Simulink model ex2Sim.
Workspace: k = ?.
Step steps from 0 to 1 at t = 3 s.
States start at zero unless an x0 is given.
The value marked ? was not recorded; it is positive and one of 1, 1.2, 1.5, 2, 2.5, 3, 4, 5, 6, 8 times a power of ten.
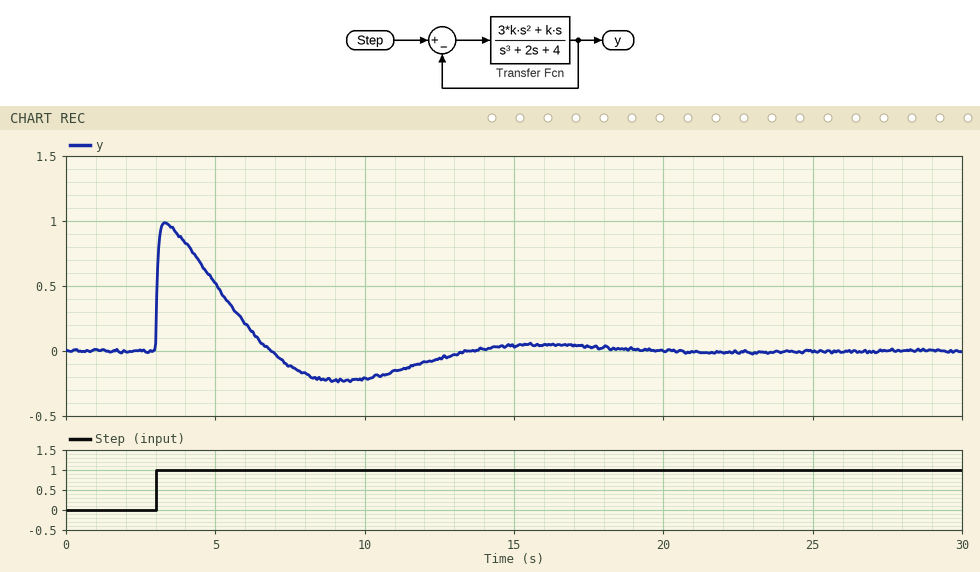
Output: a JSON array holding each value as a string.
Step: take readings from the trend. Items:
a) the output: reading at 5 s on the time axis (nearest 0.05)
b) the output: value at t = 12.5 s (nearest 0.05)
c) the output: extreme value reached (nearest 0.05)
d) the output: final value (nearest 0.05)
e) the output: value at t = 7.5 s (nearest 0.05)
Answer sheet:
["0.50", "-0.05", "1.00", "0.00", "-0.10"]
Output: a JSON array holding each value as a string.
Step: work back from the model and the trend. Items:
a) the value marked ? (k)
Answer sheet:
["5"]
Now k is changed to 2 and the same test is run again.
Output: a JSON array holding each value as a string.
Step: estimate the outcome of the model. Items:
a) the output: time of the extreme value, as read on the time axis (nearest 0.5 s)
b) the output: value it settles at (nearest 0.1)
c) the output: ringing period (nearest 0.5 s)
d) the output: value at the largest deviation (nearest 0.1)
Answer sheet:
["3.5 s", "0.0", "7.0 s", "0.9"]
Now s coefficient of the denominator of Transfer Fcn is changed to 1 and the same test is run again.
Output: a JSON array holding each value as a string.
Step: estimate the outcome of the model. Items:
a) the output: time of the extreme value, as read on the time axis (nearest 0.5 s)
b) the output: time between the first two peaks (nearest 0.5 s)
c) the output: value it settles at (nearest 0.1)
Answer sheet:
["3.5 s", "12.5 s", "0.0"]
